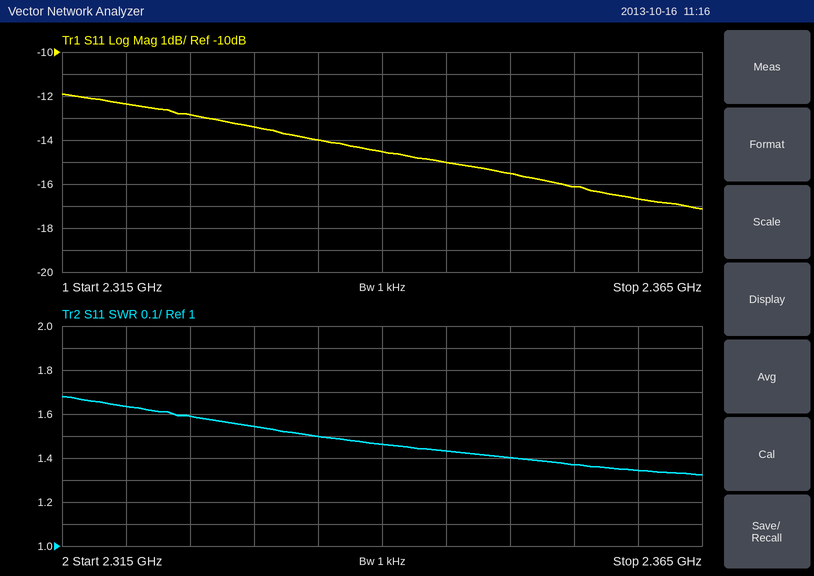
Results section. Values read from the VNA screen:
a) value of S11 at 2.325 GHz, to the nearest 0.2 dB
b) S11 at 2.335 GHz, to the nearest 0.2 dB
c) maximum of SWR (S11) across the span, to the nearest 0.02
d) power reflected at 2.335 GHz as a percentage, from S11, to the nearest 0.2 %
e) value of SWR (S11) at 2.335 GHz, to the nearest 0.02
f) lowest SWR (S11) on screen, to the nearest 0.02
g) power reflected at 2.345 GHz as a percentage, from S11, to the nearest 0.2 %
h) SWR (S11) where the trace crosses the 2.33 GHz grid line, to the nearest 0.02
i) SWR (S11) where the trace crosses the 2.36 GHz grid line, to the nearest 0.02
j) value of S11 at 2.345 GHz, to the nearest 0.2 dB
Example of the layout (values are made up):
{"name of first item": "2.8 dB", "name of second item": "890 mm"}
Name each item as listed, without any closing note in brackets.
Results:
{"value of S11 at 2.325 GHz, to the nearest 0.2 dB": "-12.8 dB", "S11 at 2.335 GHz, to the nearest 0.2 dB": "-14.0 dB", "maximum of SWR (S11) across the span, to the nearest 0.02": "1.68", "power reflected at 2.335 GHz as a percentage, from S11, to the nearest 0.2 %": "4.0 %", "value of SWR (S11) at 2.335 GHz, to the nearest 0.02": "1.50", "lowest SWR (S11) on screen, to the nearest 0.02": "1.32", "power reflected at 2.345 GHz as a percentage, from S11, to the nearest 0.2 %": "3.2 %", "SWR (S11) where the trace crosses the 2.33 GHz grid line, to the nearest 0.02": "1.54", "SWR (S11) where the trace crosses the 2.36 GHz grid line, to the nearest 0.02": "1.34", "value of S11 at 2.345 GHz, to the nearest 0.2 dB": "-15.0 dB"}
